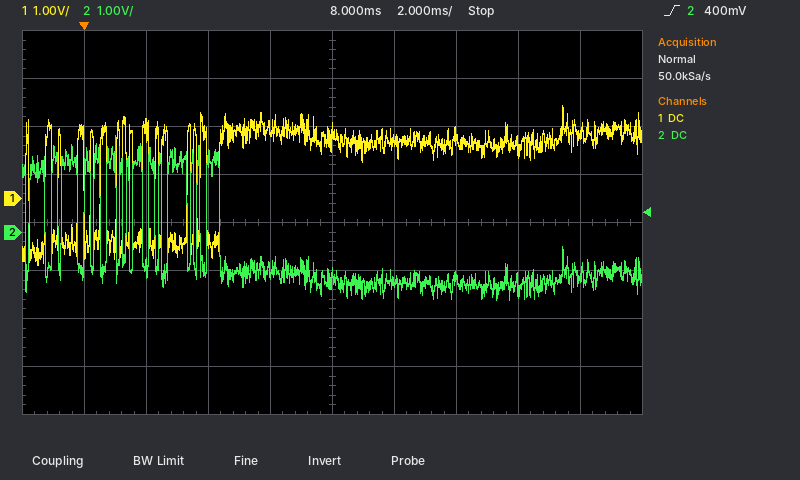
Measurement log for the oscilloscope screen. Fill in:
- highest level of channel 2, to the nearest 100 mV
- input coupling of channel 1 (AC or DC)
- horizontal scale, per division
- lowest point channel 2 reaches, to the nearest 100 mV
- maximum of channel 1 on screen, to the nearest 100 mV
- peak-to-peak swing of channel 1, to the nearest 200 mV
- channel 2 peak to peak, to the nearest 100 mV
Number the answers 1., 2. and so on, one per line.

1. 2.0 V
2. DC
3. 2 ms
4. -1.4 V
5. 1.9 V
6. 3.4 V
7. 3.4 V
